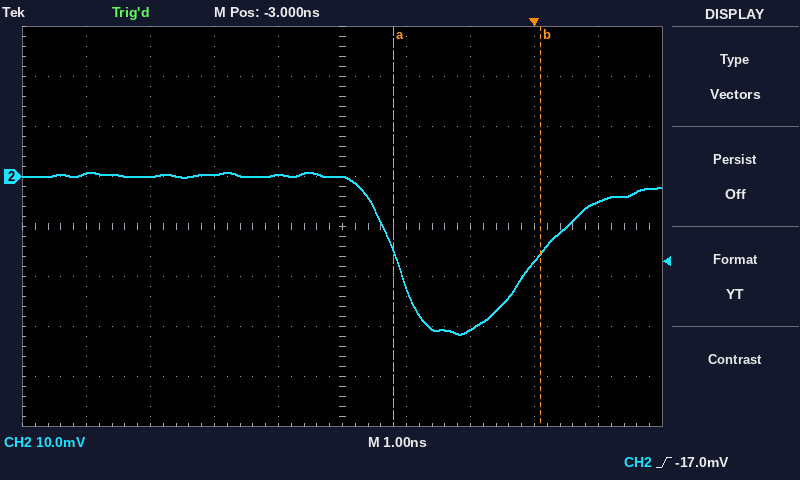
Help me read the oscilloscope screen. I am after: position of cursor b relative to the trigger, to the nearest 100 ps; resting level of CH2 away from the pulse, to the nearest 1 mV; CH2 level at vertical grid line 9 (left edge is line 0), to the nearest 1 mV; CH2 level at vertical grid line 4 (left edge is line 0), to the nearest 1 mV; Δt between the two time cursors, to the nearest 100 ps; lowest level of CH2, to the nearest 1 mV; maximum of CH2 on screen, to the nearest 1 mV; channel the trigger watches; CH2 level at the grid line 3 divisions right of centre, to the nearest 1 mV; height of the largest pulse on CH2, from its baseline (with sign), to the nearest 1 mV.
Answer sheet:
+100 ps
0 mV
-5 mV
0 mV
2.3 ns
-32 mV
1 mV
CH2
-17 mV
-32 mV
